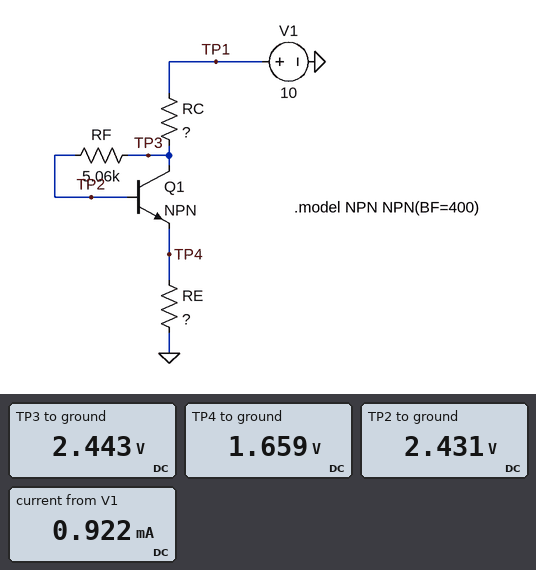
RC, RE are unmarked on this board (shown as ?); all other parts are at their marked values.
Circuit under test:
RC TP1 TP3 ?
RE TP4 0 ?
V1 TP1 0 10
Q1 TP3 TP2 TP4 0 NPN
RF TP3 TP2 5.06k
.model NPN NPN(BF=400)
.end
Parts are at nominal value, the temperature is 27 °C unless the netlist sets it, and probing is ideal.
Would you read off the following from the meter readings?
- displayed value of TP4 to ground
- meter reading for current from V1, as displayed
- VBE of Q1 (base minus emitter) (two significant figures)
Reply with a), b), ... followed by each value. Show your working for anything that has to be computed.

a) 1.659 V
b) 0.922 mA
c) 2.431 V - 1.659 V = 770 mV
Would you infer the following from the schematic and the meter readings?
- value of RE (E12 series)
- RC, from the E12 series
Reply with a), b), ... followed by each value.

a) 1.8 kΩ
b) 8.2 kΩ
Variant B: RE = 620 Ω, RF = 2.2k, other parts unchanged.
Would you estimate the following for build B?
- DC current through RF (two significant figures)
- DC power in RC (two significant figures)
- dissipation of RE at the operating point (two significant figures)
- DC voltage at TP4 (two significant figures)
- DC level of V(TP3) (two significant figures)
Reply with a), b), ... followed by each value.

a) 2.6 µA
b) 9.0 mW
c) 680 µW
d) 650 mV
e) 1.4 V
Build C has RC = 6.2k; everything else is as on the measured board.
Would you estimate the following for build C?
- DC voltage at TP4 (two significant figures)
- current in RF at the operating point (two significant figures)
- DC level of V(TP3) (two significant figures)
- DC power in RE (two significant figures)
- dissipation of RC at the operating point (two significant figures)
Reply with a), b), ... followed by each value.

a) 2.1 V
b) 2.9 µA
c) 2.9 V
d) 2.4 mW
e) 8.2 mW
